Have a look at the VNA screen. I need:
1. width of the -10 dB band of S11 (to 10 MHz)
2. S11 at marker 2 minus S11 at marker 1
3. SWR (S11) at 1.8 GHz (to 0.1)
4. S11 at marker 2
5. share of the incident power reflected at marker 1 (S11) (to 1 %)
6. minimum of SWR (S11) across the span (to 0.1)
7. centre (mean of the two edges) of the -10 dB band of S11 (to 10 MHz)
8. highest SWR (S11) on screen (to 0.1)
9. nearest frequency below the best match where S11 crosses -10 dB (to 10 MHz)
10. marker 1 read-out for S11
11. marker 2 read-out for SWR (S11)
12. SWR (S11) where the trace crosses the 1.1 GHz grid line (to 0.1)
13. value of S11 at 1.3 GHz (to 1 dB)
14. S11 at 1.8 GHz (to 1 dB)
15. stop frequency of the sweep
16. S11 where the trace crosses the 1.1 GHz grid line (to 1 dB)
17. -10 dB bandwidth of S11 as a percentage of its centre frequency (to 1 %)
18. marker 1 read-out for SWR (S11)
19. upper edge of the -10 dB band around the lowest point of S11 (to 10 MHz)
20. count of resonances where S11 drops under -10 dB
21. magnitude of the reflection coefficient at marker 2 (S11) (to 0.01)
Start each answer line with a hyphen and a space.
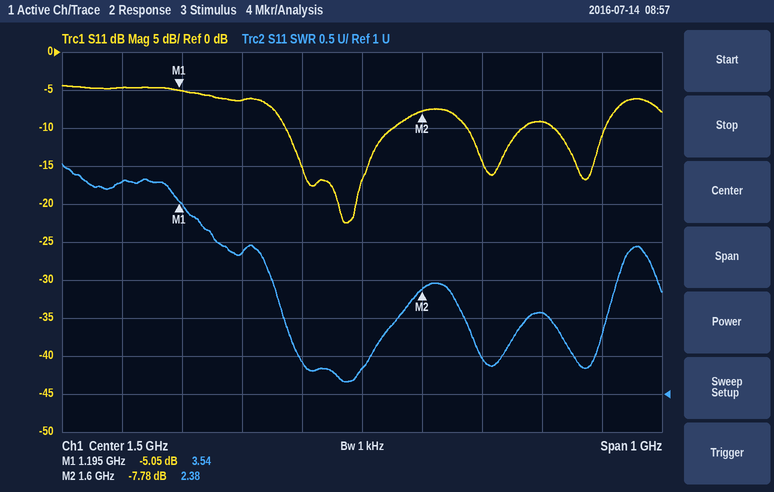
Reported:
- 180 MHz
- -2.73 dB
- 2.1
- -7.78 dB
- 31 %
- 1.2
- 1.46 GHz
- 4.0
- 1.37 GHz
- -5.05 dB
- 2.38
- 3.8
- -6 dB
- -9 dB
- 2 GHz
- -5 dB
- 12 %
- 3.54
- 1.55 GHz
- 3
- 0.41
